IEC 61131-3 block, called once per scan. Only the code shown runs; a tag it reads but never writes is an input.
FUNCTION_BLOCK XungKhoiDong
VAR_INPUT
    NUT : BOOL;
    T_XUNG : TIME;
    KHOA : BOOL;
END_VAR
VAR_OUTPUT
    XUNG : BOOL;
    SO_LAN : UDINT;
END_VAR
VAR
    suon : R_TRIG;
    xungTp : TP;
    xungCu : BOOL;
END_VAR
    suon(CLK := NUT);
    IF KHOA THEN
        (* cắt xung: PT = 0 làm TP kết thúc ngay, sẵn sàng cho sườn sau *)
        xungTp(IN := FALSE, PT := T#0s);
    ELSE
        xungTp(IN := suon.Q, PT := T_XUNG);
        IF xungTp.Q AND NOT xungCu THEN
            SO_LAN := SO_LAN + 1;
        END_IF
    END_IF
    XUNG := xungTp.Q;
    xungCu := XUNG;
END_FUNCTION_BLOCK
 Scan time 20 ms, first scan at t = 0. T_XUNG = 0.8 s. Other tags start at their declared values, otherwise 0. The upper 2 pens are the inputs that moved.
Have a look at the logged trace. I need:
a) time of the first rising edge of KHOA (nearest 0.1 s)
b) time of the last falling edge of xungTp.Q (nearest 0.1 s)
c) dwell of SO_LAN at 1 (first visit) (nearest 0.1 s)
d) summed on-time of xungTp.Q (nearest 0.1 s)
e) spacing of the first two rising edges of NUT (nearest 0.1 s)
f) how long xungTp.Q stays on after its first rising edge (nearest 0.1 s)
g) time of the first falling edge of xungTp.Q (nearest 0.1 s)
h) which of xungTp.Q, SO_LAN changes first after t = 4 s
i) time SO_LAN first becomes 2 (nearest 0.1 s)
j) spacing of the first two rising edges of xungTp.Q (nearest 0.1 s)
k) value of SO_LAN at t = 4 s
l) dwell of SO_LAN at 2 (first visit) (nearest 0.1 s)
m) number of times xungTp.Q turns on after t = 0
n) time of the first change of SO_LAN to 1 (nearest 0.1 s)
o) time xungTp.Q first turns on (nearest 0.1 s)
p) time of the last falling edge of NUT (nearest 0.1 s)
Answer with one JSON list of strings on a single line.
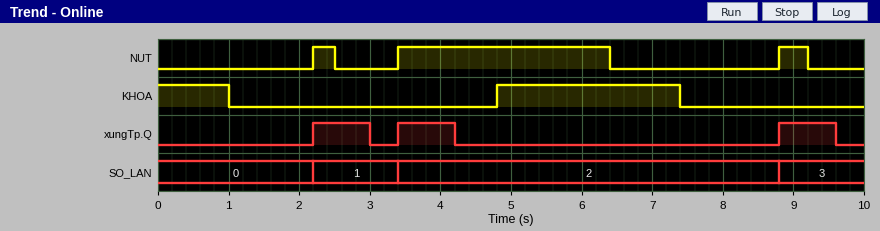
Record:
["4.8 s", "9.6 s", "1.2 s", "2.4 s", "1.2 s", "0.8 s", "3.0 s", "xungTp.Q", "3.4 s", "1.2 s", "2", "5.4 s", "3", "2.2 s", "2.2 s", "9.2 s"]
